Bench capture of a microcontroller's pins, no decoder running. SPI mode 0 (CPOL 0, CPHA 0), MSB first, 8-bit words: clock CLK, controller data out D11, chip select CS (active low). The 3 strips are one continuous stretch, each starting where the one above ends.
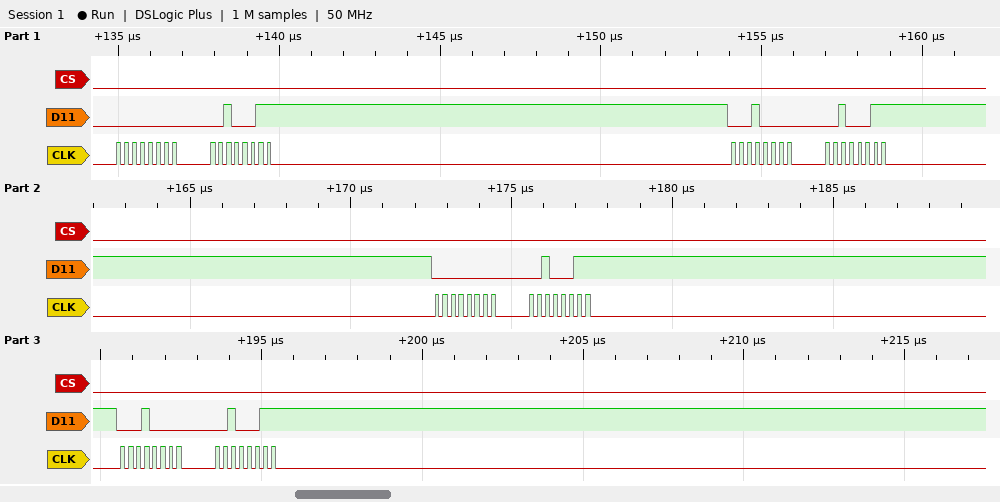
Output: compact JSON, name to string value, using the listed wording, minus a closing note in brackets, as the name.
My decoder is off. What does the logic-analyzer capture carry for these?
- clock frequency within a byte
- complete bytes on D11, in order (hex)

{"clock frequency within a byte": "4 MHz", "complete bytes on D11, in order": "00 23 10 23 00 23 10 23"}
